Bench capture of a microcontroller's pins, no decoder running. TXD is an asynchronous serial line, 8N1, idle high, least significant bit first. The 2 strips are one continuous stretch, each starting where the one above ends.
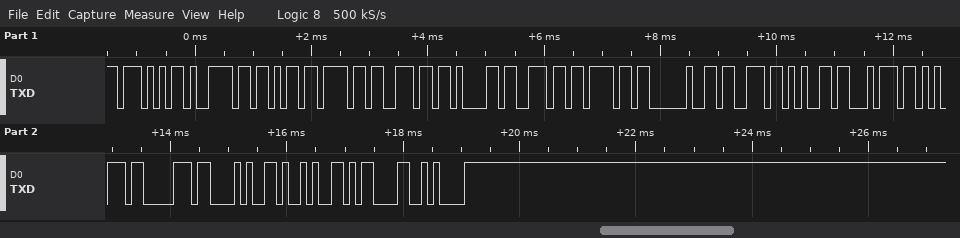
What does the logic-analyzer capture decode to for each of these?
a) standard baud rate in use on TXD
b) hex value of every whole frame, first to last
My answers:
9600 baud
0x57 0x79 0x6B 0x6F 0x6E 0x61 0x6E 0x6F 0x20 0x73 0x65 0x74 0x75 0x70 0x28 0x29 0x0D 0x0A
